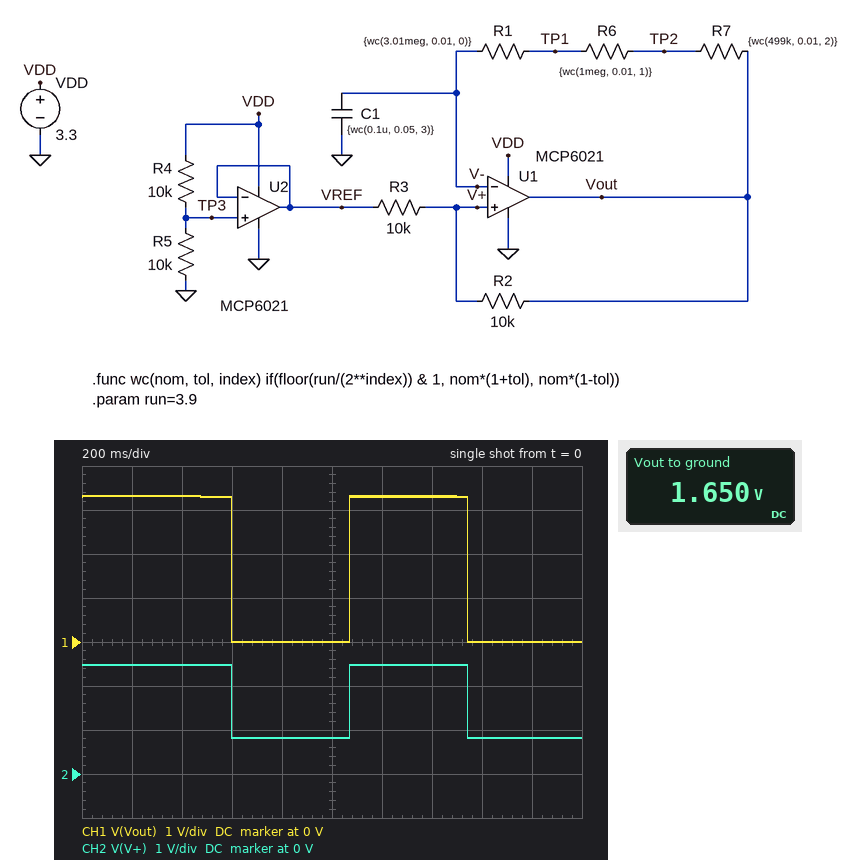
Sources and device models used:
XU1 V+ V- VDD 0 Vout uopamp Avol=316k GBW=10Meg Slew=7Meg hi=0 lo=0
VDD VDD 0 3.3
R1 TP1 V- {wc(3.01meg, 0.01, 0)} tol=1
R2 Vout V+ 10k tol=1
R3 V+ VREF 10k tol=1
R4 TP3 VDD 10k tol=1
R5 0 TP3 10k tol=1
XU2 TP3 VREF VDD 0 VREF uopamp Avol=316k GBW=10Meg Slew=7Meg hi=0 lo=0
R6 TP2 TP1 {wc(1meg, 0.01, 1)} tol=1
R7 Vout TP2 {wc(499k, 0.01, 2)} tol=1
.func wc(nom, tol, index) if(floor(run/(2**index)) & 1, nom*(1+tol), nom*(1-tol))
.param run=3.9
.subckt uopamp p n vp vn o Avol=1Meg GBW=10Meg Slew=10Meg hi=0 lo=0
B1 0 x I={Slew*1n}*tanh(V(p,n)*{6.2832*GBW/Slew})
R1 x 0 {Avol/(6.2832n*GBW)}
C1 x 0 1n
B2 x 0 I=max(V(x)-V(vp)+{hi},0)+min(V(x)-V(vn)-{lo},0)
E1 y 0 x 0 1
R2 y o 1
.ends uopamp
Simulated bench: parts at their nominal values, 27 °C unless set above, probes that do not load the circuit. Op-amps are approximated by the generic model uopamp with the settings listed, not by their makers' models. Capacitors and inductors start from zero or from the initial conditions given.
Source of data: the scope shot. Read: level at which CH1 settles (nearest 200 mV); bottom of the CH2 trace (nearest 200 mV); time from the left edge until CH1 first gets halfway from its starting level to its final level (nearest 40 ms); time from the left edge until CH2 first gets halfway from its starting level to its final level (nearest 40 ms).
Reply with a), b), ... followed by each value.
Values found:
a) 0 V
b) 800 mV
c) 600 ms
d) 600 ms
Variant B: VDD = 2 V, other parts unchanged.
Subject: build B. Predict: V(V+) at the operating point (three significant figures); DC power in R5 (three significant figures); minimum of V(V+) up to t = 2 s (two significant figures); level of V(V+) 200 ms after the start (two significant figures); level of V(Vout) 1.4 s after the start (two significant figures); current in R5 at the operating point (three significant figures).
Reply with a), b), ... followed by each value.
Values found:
a) 1.00 V
b) 100 µW
c) 500 mV
d) 1.5 V
e) 2.0 V
f) 100 µA
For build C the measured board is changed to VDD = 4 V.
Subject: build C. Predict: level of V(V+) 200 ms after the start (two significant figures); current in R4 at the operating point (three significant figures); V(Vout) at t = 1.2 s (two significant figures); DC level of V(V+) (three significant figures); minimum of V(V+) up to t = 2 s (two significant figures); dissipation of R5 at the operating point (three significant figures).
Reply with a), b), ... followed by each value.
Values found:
a) 3.0 V
b) 200 µA
c) 4.0 V
d) 2.00 V
e) 1.0 V
f) 400 µW
